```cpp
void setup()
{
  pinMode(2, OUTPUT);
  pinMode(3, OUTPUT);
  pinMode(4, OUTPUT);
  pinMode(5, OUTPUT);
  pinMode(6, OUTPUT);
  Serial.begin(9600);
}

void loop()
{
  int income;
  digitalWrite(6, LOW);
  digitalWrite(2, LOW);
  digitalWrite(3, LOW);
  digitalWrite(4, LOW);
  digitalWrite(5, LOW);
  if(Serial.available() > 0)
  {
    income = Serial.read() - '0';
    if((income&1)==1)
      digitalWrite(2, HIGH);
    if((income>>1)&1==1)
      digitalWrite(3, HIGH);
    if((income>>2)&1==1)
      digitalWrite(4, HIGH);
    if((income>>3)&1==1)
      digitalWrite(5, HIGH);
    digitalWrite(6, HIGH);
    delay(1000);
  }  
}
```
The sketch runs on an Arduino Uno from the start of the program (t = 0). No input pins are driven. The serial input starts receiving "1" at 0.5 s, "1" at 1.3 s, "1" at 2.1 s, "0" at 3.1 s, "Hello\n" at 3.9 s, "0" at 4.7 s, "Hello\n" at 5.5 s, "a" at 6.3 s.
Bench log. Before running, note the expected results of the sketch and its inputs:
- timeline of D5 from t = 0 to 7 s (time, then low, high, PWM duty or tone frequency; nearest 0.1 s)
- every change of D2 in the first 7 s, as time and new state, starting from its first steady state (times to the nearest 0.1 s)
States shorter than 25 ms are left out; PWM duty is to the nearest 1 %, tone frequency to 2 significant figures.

0 s low; 4.5 s high; 5.5 s low; 6.5 s high
0 s low; 0.5 s high; 3.5 s low; 5.5 s high; 6.5 s low
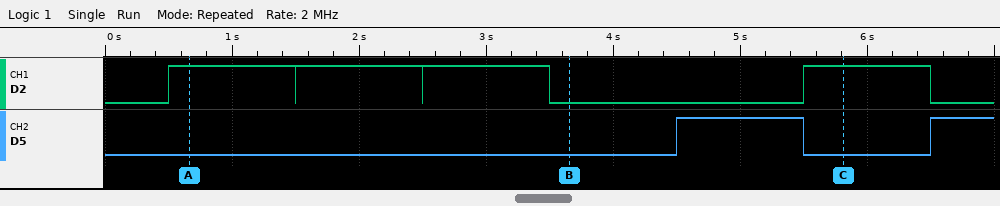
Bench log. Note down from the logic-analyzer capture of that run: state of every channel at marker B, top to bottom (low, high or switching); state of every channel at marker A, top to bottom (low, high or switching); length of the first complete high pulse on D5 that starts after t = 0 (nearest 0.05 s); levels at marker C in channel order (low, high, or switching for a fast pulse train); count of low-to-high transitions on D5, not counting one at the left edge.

D2 low, D5 low
D2 high, D5 low
1.00 s
D2 high, D5 low
2
